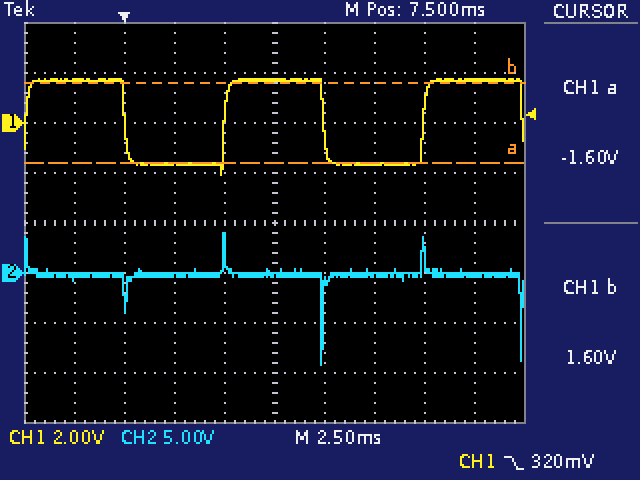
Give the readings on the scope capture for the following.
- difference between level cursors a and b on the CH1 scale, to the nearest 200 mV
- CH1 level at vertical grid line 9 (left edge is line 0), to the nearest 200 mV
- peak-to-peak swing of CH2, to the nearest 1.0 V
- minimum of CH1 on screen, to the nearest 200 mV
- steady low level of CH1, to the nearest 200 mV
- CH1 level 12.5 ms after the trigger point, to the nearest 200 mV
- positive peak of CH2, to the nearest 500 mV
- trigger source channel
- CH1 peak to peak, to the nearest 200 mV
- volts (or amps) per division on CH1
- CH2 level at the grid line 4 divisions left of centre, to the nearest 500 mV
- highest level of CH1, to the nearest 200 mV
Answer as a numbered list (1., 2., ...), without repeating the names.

1. 3.2 V
2. 1.8 V
3. 13.0 V
4. -2.0 V
5. -1.6 V
6. -1.6 V
7. 4.0 V
8. CH1
9. 3.8 V
10. 2 V
11. -500 mV
12. 1.8 V
